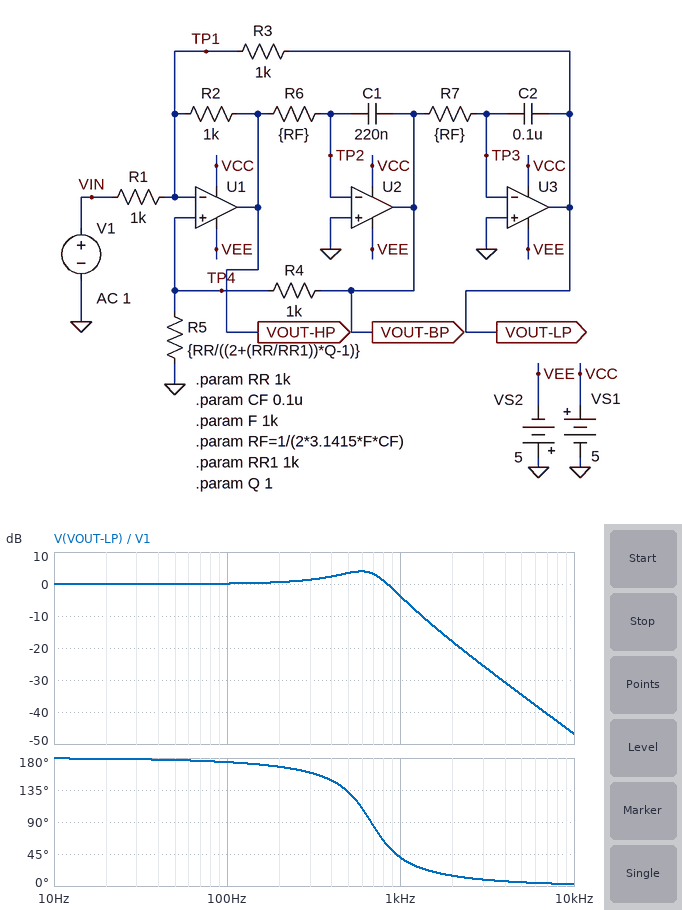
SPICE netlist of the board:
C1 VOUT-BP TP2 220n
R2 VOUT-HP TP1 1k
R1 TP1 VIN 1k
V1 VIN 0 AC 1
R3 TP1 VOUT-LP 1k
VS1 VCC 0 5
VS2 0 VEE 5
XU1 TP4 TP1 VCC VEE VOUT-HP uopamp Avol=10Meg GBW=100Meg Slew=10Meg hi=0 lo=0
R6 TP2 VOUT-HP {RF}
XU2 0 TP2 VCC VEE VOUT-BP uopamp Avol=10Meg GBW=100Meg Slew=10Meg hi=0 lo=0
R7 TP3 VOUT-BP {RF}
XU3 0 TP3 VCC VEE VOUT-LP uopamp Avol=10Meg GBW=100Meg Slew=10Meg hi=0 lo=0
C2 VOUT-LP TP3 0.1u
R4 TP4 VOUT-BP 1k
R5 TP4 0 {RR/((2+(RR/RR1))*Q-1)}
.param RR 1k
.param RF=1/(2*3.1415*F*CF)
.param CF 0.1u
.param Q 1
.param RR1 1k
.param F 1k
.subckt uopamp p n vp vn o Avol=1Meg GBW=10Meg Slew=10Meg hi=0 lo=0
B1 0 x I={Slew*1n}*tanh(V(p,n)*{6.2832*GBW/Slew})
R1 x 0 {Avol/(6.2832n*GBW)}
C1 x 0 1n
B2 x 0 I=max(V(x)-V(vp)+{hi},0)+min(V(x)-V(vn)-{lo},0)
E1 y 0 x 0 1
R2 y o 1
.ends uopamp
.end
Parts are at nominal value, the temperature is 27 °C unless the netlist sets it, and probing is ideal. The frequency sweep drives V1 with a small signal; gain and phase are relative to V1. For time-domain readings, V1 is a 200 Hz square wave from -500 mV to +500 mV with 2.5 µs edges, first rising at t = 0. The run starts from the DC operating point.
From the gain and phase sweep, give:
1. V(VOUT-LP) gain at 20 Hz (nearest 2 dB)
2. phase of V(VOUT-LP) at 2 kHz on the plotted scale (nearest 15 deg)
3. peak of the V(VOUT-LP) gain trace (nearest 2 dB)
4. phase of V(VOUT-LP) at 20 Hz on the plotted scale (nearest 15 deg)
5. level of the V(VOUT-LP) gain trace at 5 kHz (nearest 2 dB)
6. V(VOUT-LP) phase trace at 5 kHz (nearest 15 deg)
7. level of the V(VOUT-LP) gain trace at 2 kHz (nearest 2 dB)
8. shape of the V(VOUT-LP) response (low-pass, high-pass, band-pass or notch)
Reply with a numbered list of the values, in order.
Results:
1. 0 dB
2. 15 deg
3. 4 dB
4. 180 deg
5. -34 dB
6. 0 deg
7. -18 dB
8. low-pass
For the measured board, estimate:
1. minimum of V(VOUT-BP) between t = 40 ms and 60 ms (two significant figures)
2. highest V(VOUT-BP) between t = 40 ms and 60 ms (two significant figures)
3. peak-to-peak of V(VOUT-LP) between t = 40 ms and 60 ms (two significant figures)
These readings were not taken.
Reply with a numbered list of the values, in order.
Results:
1. -450 mV
2. 450 mV
3. 1.7 V
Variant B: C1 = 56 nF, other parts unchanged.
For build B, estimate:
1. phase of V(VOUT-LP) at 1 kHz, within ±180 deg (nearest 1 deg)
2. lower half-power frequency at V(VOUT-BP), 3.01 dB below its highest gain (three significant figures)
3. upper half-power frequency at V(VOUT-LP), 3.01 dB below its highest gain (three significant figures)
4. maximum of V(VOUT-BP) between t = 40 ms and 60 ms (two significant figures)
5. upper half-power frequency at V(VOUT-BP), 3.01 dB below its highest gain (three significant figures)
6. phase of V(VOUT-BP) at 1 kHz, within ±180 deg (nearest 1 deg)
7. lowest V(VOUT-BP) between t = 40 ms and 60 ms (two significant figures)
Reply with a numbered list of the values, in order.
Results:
1. 114 deg
2. 714 Hz
3. 1.40 kHz
4. 630 mV
5. 2.50 kHz
6. 24 deg
7. -630 mV
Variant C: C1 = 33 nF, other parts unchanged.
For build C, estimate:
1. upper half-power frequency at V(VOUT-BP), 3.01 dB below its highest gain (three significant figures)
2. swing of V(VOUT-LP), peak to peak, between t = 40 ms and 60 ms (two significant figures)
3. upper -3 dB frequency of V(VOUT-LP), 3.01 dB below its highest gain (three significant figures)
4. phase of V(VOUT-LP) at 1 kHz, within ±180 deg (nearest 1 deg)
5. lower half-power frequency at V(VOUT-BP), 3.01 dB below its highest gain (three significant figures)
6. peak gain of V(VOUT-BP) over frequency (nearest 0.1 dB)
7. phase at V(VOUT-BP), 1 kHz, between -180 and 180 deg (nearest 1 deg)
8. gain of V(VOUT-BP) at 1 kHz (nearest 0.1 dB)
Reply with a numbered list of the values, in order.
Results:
1. 3.82 kHz
2. 1.0 V
3. 1.36 kHz
4. 124 deg
5. 793 Hz
6. 0 dB
7. 34 deg
8. -1.6 dB
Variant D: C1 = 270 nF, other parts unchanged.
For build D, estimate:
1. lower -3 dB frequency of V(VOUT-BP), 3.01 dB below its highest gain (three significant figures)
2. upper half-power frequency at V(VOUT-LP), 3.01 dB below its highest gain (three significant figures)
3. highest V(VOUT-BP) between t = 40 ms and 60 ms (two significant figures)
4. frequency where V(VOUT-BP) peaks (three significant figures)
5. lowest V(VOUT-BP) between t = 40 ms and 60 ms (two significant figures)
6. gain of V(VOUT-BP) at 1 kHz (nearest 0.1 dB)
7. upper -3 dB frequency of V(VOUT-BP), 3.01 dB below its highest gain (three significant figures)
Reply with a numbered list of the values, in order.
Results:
1. 451 Hz
2. 719 Hz
3. 430 mV
4. 609 Hz
5. -430 mV
6. -5.9 dB
7. 821 Hz
